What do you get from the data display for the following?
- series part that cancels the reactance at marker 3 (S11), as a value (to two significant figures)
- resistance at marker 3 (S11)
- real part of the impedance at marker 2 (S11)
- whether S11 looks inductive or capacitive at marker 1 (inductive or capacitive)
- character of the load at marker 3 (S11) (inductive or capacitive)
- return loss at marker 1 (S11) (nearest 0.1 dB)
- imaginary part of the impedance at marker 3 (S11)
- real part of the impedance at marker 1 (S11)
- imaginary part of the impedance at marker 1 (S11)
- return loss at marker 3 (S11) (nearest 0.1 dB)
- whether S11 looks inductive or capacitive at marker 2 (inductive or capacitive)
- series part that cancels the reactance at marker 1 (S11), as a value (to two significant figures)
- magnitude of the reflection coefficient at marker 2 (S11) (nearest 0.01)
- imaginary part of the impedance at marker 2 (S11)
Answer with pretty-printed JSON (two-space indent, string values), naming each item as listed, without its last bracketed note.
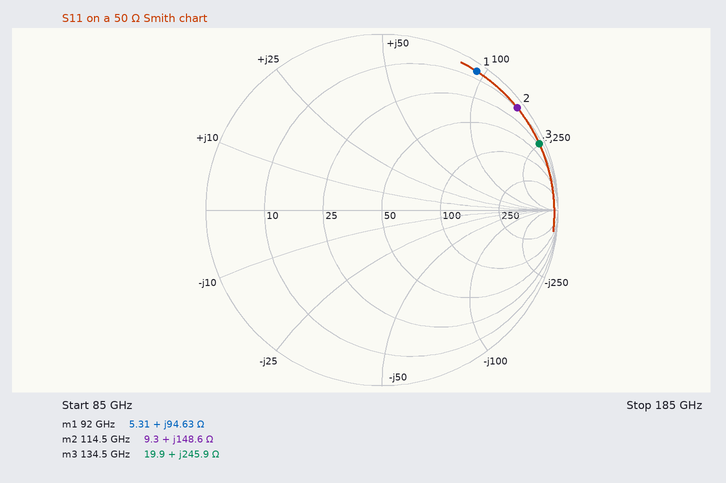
{
  "series part that cancels the reactance at marker 3 (S11), as a value": "4.8 fF",
  "resistance at marker 3": "19.9 Ω",
  "real part of the impedance at marker 2": "9.3 Ω",
  "whether S11 looks inductive or capacitive at marker 1": "inductive",
  "character of the load at marker 3 (S11)": "inductive",
  "return loss at marker 1 (S11)": "0.4 dB",
  "imaginary part of the impedance at marker 3": "+245.9 Ω",
  "real part of the impedance at marker 1": "5.31 Ω",
  "imaginary part of the impedance at marker 1": "+94.63 Ω",
  "return loss at marker 3 (S11)": "0.3 dB",
  "whether S11 looks inductive or capacitive at marker 2": "inductive",
  "series part that cancels the reactance at marker 1 (S11), as a value": "18 fF",
  "magnitude of the reflection coefficient at marker 2 (S11)": "0.96",
  "imaginary part of the impedance at marker 2": "+148.6 Ω"
}
